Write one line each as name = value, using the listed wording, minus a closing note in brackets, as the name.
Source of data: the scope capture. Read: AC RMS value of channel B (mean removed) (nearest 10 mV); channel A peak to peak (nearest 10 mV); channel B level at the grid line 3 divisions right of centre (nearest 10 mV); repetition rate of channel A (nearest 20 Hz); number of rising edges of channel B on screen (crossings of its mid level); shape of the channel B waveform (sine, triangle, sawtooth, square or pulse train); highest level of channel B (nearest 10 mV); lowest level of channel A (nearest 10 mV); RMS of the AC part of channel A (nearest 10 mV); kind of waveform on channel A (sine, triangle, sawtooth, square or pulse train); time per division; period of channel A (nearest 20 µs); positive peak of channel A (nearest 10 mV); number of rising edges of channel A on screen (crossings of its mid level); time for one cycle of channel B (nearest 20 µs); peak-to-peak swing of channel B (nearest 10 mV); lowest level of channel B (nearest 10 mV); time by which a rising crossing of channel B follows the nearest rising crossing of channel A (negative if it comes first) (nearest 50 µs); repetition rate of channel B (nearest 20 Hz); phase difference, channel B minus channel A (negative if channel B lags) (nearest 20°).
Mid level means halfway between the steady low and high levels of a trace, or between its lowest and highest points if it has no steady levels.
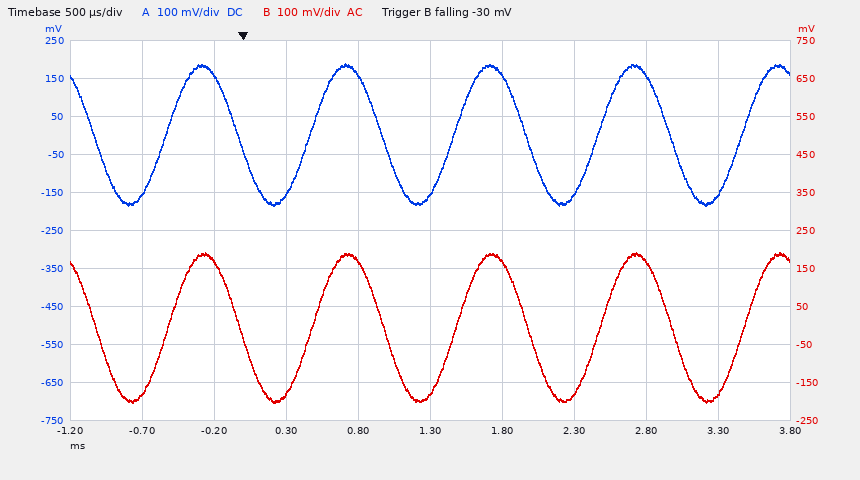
AC RMS value of channel B (mean removed) = 140 mV
channel A peak to peak = 370 mV
channel B level at the grid line 3 divisions right of centre = 170 mV
repetition rate of channel A = 1.00 kHz
number of rising edges of channel B on screen = 5
shape of the channel B waveform = sine
highest level of channel B = 190 mV
lowest level of channel A = -180 mV
RMS of the AC part of channel A = 130 mV
kind of waveform on channel A = sine
time per division = 500 µs
period of channel A = 1.00 ms
positive peak of channel A = 190 mV
number of rising edges of channel A on screen = 5
time for one cycle of channel B = 1.00 ms
peak-to-peak swing of channel B = 390 mV
lowest level of channel B = -200 mV
time by which a rising crossing of channel B follows the nearest rising crossing of channel A (negative if it comes first) = 0 µs
repetition rate of channel B = 1.00 kHz
phase difference, channel B minus channel A (negative if channel B lags) = 0°
